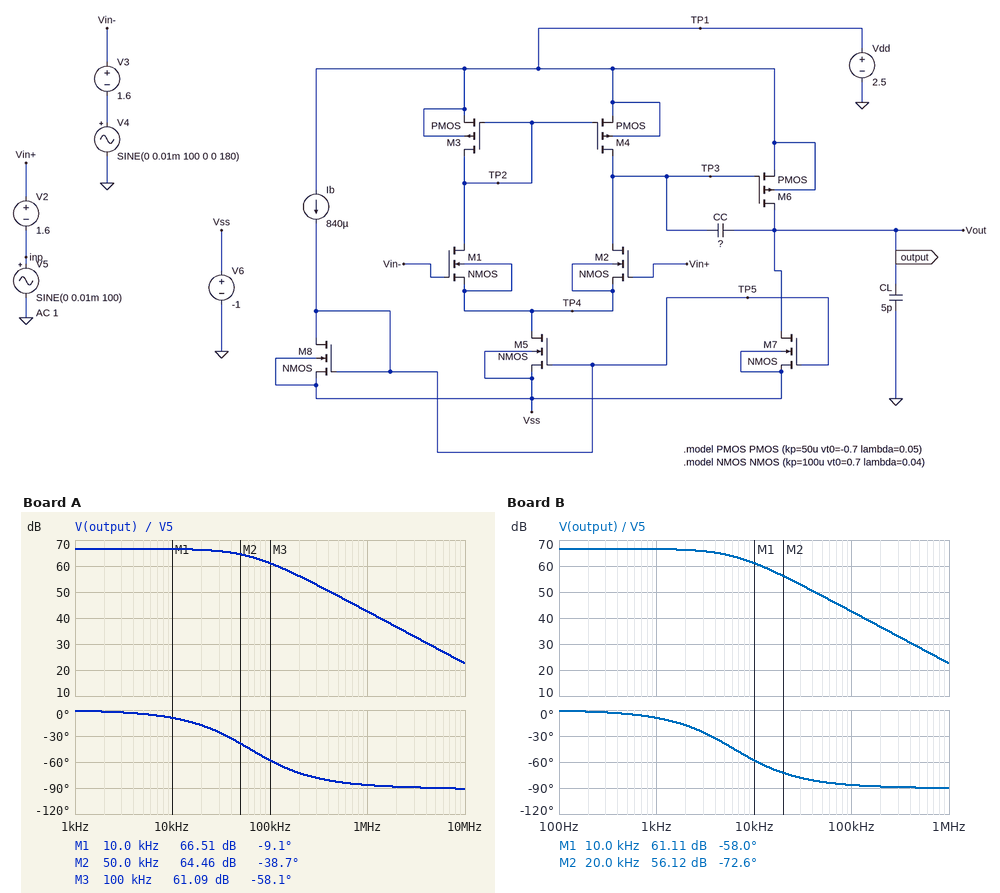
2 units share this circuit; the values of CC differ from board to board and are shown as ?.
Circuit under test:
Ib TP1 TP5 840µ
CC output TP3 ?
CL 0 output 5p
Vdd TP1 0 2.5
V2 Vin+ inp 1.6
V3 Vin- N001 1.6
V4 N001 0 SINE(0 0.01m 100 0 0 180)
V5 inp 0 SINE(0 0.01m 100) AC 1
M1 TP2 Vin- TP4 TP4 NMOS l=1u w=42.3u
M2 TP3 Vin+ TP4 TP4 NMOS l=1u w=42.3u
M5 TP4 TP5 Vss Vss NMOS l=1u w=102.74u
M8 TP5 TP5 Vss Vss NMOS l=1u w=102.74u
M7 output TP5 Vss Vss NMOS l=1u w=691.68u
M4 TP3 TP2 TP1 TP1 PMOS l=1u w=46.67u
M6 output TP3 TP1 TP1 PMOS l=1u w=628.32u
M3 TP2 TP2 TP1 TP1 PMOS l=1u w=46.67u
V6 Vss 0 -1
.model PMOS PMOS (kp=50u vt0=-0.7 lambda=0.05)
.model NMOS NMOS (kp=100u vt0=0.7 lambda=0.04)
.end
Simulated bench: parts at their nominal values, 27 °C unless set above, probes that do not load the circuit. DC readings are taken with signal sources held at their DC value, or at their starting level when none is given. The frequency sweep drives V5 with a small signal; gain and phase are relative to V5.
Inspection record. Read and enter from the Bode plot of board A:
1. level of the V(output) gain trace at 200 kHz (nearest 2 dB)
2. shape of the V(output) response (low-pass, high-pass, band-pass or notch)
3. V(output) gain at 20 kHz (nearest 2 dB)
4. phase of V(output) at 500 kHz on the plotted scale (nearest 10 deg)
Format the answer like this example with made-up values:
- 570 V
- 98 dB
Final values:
- 56 dB
- low-pass
- 66 dB
- -80 deg
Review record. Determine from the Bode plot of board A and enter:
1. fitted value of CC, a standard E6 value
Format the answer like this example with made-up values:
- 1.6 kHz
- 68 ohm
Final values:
- 2.2 pF
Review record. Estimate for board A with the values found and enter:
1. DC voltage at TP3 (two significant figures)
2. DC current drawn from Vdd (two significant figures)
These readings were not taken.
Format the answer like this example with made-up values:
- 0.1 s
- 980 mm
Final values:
- 1.2 V
- 7.5 mA
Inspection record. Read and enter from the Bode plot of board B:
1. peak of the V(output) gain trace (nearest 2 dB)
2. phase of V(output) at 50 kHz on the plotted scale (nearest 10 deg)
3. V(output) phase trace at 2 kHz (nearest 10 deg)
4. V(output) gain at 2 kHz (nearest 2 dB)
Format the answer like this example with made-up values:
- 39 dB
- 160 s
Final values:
- 66 dB
- -80 deg
- -20 deg
- 66 dB
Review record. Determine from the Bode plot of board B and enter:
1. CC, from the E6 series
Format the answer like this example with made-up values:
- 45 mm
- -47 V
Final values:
- 22 pF
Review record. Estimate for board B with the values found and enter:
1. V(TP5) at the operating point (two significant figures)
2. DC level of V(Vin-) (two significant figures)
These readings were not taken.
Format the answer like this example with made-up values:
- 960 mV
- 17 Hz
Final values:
- 96 mV
- 1.6 V
